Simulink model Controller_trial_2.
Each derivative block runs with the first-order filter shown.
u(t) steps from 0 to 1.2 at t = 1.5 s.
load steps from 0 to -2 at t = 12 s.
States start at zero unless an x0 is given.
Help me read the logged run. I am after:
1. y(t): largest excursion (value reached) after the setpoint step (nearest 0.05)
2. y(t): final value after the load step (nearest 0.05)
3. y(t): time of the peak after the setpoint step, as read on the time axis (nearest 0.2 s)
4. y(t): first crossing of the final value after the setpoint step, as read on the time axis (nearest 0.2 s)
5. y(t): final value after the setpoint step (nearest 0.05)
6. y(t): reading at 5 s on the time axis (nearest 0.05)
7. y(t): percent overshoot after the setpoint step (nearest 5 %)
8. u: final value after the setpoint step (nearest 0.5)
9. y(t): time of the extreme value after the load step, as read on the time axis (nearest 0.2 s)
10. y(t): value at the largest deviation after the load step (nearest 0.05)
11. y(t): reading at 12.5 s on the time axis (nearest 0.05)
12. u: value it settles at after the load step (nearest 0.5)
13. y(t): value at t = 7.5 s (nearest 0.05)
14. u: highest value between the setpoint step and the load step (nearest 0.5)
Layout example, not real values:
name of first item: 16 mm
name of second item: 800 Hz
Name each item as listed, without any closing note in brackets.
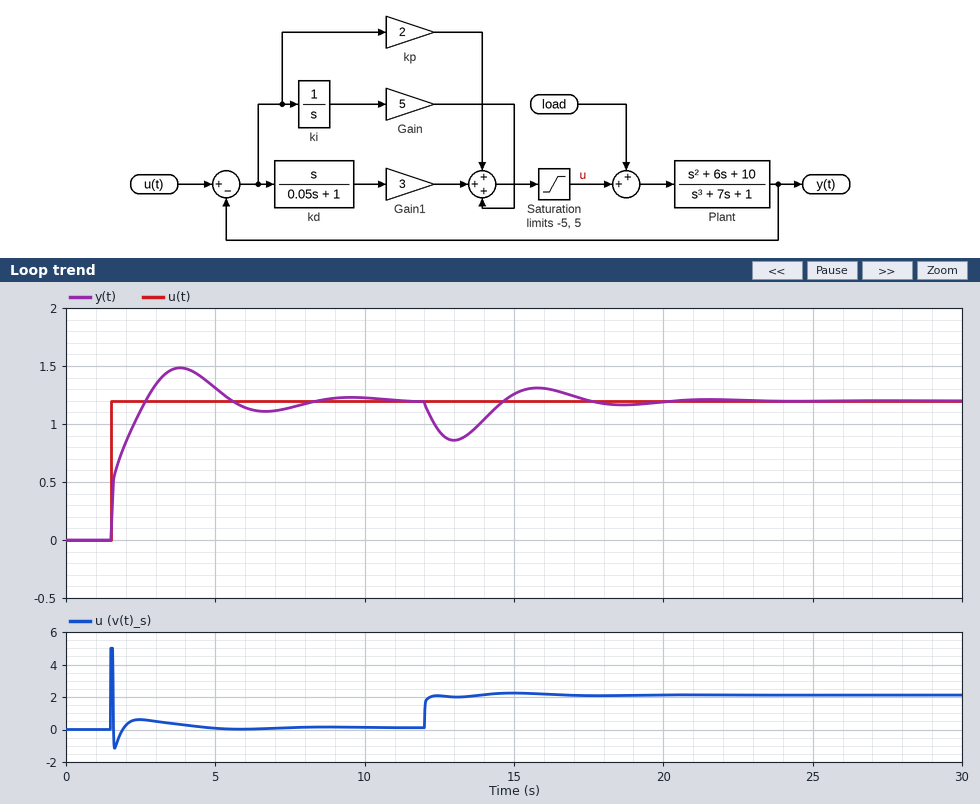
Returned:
y(t): largest excursion (value reached) after the setpoint step: 1.50
y(t): final value after the load step: 1.20
y(t): time of the peak after the setpoint step, as read on the time axis: 3.8 s
y(t): first crossing of the final value after the setpoint step, as read on the time axis: 2.6 s
y(t): final value after the setpoint step: 1.20
y(t): reading at 5 s on the time axis: 1.30
y(t): percent overshoot after the setpoint step: 25 %
u: final value after the setpoint step: 0.0
y(t): time of the extreme value after the load step, as read on the time axis: 13.0 s
y(t): value at the largest deviation after the load step: 0.85
y(t): reading at 12.5 s on the time axis: 0.95
u: value it settles at after the load step: 2.0
y(t): value at t = 7.5 s: 1.15
u: highest value between the setpoint step and the load step: 5.0
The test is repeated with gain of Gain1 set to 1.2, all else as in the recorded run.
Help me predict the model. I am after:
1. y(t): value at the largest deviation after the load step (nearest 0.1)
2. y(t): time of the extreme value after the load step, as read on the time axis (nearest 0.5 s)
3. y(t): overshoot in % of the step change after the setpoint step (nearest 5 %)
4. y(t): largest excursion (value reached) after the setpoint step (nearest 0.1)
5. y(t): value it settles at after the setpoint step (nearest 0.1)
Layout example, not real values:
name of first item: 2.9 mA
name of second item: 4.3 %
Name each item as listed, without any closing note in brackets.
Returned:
y(t): value at the largest deviation after the load step: 0.7
y(t): time of the extreme value after the load step, as read on the time axis: 12.5 s
y(t): overshoot in % of the step change after the setpoint step: 10 %
y(t): largest excursion (value reached) after the setpoint step: 1.3
y(t): value it settles at after the setpoint step: 1.2
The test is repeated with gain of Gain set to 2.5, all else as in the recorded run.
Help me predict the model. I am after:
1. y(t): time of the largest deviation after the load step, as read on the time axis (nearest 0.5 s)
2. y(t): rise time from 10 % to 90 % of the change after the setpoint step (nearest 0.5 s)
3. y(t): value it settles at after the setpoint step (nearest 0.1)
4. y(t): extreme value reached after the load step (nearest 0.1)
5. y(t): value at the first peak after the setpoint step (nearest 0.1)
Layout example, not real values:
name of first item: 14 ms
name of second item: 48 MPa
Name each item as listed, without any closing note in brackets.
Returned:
y(t): time of the largest deviation after the load step, as read on the time axis: 13.5 s
y(t): rise time from 10 % to 90 % of the change after the setpoint step: 1.5 s
y(t): value it settles at after the setpoint step: 1.2
y(t): extreme value reached after the load step: 0.8
y(t): value at the first peak after the setpoint step: 1.4
